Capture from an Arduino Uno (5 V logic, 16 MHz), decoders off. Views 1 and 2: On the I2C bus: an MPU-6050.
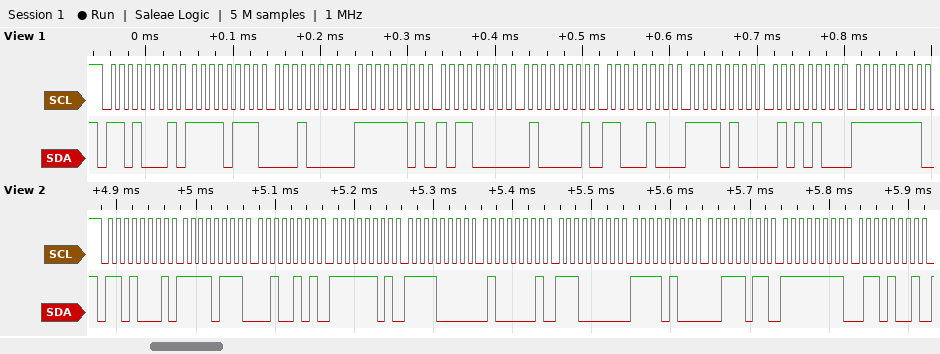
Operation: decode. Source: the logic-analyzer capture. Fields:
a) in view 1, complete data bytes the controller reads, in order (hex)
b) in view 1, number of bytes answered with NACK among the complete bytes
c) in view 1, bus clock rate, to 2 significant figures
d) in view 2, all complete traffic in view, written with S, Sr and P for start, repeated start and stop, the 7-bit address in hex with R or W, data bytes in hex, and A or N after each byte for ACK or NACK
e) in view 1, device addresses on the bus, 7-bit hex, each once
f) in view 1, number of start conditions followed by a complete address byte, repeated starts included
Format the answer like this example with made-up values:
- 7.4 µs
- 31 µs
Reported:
- F7 10 FD B0 41 C4 F4 54 FF
- 0
- 100 kHz
- S 68R A F7 A 25 A FD A F0 A 41 A E0 A F4 A 3B A FF A 69 A
- 0x68
- 1
